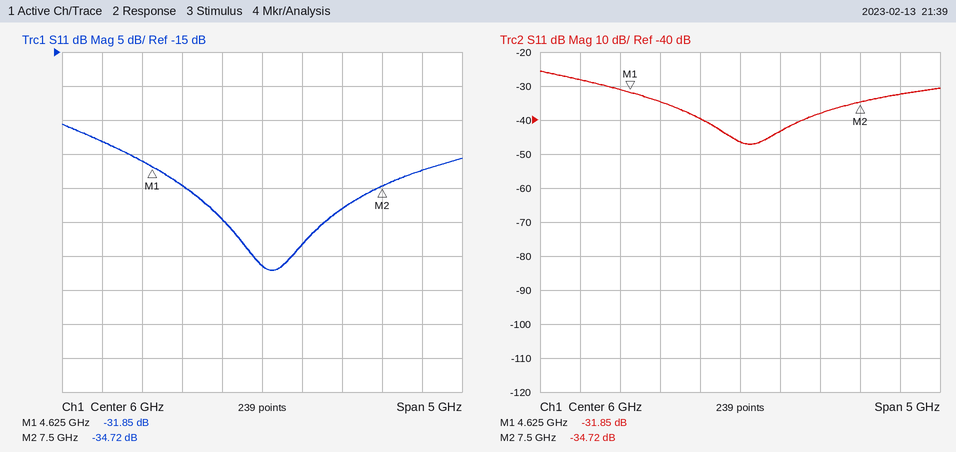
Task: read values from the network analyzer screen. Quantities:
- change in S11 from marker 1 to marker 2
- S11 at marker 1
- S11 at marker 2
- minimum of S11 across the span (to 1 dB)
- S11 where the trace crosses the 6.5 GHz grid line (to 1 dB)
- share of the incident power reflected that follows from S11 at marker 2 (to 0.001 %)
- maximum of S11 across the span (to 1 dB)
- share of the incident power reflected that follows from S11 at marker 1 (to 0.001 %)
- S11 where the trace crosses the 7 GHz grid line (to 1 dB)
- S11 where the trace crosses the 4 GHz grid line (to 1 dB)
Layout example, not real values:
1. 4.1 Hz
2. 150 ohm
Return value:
1. -2.87 dB
2. -31.85 dB
3. -34.72 dB
4. -47 dB
5. -43 dB
6. 0.034 %
7. -26 dB
8. 0.065 %
9. -38 dB
10. -28 dB
